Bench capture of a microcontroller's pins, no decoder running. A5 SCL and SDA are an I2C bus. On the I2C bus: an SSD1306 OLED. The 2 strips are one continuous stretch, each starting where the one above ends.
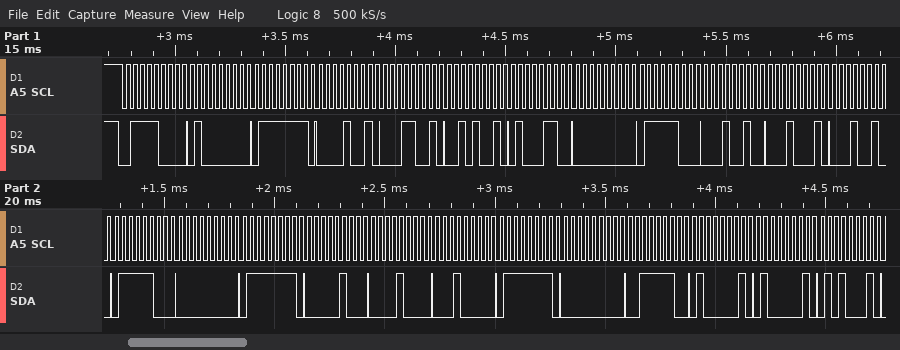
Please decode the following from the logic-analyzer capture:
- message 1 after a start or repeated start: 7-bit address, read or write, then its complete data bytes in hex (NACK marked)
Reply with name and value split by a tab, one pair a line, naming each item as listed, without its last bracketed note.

message 1 after a start or repeated start: 7-bit address, read or write, then its complete data bytes in hex	0x3C write: 40 7F 09 19 29 46 00 7C 12 11 12 7C 00 7F 04 08 10 7F 00 3E 41 41 51
